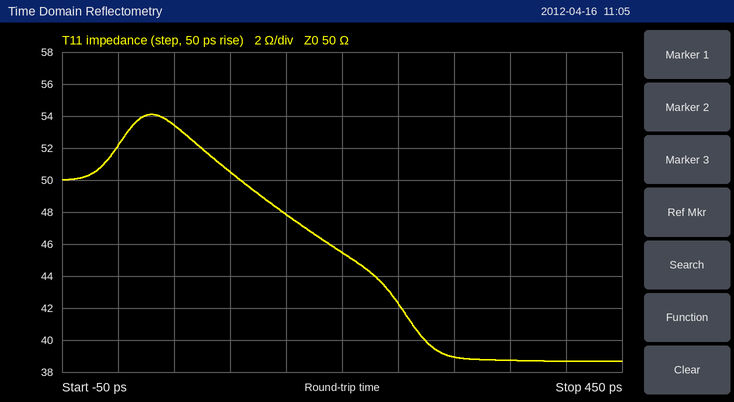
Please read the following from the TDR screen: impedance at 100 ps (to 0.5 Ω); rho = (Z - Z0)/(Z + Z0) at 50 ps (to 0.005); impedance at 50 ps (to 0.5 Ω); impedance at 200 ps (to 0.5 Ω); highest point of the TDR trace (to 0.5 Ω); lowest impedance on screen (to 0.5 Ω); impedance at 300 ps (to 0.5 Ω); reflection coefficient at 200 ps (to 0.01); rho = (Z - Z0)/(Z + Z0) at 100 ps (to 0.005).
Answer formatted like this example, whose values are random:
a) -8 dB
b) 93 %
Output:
a) 50.5 Ω
b) +0.035
c) 53.5 Ω
d) 45.5 Ω
e) 54.0 Ω
f) 38.5 Ω
g) 39.0 Ω
h) -0.05
i) +0.005
